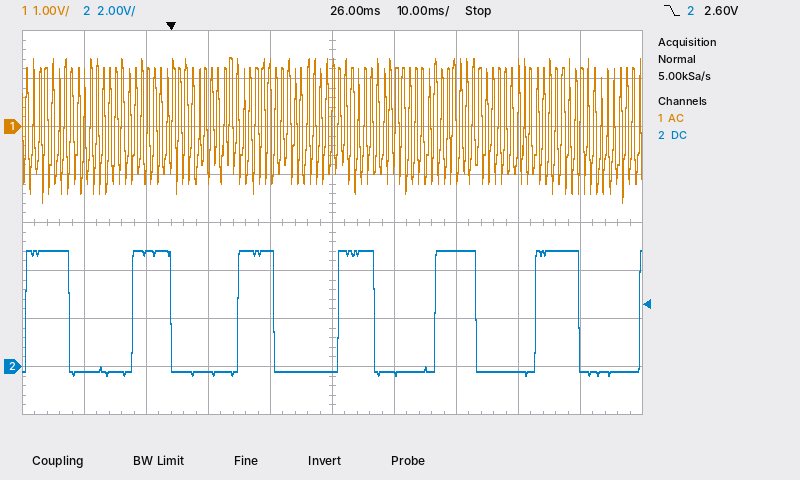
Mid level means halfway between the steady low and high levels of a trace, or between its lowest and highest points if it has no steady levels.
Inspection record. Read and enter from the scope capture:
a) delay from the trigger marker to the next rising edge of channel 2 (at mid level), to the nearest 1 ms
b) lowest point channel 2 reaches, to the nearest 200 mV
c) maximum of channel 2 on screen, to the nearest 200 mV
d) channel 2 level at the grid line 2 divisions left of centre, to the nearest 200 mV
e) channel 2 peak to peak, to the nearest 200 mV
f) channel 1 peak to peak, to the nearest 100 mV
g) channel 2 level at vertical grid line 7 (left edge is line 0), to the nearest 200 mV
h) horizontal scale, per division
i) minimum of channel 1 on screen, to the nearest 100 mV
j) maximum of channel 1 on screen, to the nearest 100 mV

11 ms
-400 mV
4.8 V
-200 mV
5.2 V
3.0 V
4.8 V
10 ms
-1.6 V
1.4 V
